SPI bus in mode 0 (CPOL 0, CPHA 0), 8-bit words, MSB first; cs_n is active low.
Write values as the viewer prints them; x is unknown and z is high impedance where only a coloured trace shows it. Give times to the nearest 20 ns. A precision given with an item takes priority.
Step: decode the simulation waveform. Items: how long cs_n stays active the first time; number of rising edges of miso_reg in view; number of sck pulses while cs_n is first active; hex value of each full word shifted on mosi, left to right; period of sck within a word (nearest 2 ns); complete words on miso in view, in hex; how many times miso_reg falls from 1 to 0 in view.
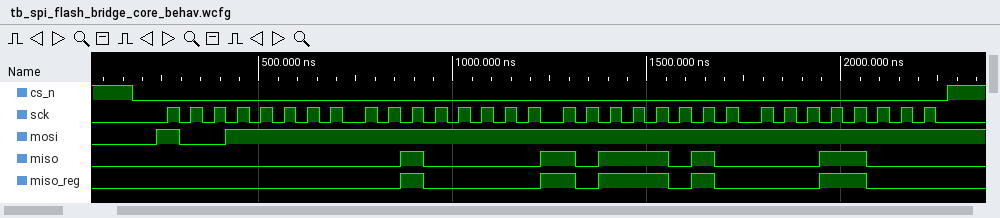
2100 ns
5
32
9F, FF, FF, FF
60 ns
00, 20, BA, 18
5
